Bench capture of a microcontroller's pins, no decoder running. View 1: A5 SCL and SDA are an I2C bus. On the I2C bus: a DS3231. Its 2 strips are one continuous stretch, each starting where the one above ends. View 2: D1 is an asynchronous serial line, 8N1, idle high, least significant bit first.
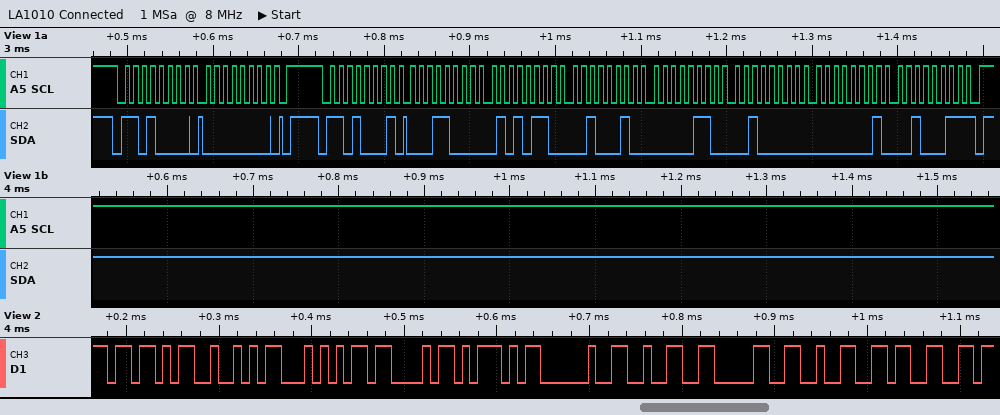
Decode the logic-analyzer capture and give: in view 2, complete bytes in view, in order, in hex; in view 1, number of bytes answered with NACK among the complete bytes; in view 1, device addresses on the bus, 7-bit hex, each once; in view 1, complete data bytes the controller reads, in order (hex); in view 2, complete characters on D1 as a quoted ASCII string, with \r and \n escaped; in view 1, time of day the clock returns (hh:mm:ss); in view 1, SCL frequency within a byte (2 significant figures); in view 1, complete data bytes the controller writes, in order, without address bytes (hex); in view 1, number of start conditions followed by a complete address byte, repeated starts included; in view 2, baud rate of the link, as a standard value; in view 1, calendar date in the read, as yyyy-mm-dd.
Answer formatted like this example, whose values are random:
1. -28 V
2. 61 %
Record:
1. 5B 52 54 43 5D 20 32 30 32 33
2. 1
3. 0x68
4. 18 56 22 06 20 01 23
5. "[RTC] 2023"
6. 22:56:18
7. 100 kHz
8. 00
9. 2
10. 115200 baud
11. 2023-01-20
